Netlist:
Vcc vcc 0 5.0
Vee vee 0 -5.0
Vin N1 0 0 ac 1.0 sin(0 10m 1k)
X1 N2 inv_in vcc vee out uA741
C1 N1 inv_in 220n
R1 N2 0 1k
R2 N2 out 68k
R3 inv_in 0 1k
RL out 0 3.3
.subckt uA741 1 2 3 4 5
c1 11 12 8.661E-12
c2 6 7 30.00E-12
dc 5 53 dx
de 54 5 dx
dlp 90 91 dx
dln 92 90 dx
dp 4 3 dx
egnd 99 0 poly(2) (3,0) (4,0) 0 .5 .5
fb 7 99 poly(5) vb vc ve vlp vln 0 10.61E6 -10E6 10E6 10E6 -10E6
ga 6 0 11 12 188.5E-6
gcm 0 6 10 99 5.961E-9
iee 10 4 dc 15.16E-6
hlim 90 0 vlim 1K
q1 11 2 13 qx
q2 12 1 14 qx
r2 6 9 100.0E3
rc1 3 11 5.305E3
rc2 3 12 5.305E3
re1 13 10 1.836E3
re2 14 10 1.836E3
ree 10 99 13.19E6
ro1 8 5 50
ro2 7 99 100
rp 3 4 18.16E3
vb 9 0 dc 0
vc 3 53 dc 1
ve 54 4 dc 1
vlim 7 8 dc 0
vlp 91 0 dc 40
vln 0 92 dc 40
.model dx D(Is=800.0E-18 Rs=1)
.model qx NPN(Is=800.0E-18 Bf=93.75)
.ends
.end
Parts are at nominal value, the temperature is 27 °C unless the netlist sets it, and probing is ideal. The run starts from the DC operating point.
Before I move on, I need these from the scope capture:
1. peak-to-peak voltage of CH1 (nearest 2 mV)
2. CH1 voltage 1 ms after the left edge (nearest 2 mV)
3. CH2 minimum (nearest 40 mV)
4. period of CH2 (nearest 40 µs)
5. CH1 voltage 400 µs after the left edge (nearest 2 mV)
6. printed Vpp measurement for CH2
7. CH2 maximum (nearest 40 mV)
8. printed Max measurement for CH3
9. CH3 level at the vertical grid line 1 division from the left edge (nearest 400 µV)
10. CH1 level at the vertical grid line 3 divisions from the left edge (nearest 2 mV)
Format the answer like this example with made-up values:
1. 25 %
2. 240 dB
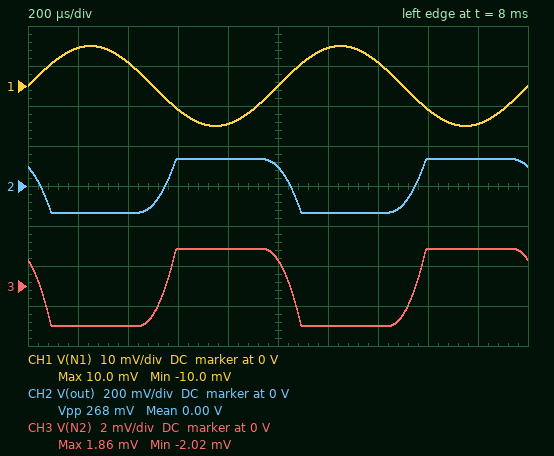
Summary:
1. 20 mV
2. 0 V
3. -120 mV
4. 1.00 ms
5. 6 mV
6. 268 mV
7. 120 mV
8. 1.86 mV
9. -2.0 mV
10. -6 mV
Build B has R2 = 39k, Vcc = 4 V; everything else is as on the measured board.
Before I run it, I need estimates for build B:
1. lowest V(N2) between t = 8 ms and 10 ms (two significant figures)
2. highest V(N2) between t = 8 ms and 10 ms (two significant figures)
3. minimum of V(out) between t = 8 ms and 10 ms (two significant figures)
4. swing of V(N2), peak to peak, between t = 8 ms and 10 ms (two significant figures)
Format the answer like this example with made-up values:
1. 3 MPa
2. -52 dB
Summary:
1. -3.4 mV
2. 3.3 mV
3. -130 mV
4. 6.7 mV
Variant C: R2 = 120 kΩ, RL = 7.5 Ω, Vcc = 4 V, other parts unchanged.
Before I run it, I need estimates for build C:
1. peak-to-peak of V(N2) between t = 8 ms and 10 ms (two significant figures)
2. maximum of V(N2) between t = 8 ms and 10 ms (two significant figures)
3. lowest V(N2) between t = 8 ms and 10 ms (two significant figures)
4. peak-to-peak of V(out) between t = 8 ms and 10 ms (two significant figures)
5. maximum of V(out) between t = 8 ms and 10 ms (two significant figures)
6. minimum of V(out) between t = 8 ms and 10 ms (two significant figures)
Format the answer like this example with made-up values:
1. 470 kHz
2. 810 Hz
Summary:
1. 5.0 mV
2. 2.4 mV
3. -2.6 mV
4. 610 mV
5. 300 mV
6. -300 mV
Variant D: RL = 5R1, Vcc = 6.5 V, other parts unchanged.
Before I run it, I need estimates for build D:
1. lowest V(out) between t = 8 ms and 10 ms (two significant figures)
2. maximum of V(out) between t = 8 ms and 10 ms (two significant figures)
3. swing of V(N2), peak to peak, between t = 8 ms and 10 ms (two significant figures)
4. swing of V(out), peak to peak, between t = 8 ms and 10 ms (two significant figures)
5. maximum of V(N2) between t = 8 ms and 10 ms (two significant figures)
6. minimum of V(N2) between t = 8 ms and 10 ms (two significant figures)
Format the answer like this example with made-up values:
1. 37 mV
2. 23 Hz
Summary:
1. -210 mV
2. 210 mV
3. 6.0 mV
4. 410 mV
5. 2.9 mV
6. -3.1 mV
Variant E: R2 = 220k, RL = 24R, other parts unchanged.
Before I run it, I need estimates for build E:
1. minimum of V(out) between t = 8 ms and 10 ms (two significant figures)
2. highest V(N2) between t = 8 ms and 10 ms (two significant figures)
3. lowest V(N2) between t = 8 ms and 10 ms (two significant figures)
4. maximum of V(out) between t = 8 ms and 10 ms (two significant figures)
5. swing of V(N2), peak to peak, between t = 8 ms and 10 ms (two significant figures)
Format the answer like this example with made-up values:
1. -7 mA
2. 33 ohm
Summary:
1. -970 mV
2. 4.3 mV
3. -4.5 mV
4. 970 mV
5. 8.8 mV
